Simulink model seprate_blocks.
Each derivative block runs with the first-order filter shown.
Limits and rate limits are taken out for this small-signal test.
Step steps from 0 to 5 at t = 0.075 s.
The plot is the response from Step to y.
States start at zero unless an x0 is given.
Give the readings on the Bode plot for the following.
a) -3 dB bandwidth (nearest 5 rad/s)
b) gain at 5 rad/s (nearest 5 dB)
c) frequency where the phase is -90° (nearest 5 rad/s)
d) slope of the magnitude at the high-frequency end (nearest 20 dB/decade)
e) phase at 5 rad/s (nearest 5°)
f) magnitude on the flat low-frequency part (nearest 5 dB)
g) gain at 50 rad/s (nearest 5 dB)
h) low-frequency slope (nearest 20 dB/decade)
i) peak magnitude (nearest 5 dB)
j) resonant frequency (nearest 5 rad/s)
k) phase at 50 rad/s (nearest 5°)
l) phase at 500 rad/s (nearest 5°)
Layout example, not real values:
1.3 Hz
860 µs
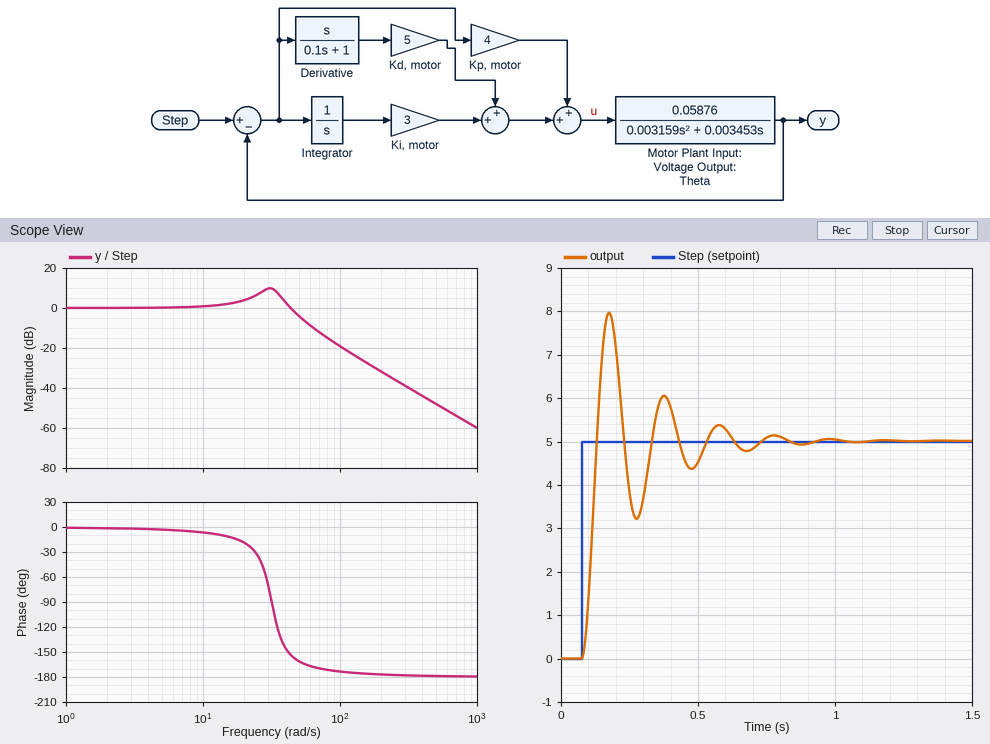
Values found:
50 rad/s
0 dB
30 rad/s
-40 dB/decade
-5°
0 dB
-5 dB
0 dB/decade
10 dB
30 rad/s
-160°
-180°
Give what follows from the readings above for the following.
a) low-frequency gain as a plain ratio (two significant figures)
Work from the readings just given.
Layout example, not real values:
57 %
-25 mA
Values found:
1.0
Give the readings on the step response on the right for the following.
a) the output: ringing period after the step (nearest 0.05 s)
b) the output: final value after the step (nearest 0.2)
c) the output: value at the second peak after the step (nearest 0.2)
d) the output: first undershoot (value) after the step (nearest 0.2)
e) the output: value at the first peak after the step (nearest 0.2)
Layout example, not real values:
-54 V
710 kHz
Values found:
0.20 s
5.0
6.0
3.2
8.0
